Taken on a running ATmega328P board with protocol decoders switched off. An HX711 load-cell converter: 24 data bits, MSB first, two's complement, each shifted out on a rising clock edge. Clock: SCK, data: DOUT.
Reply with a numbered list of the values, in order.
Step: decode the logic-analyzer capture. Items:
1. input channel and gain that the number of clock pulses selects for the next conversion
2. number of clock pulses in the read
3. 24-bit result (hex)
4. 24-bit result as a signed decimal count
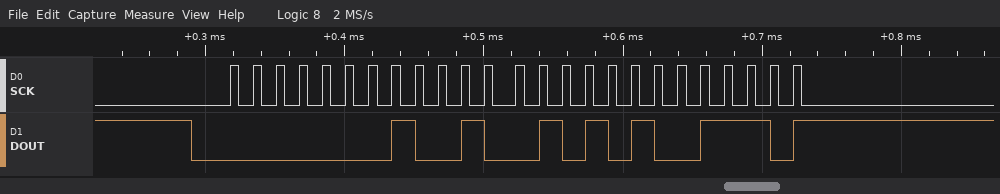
1. channel A, gain 128
2. 25
3. 0x01254E
4. 75086
